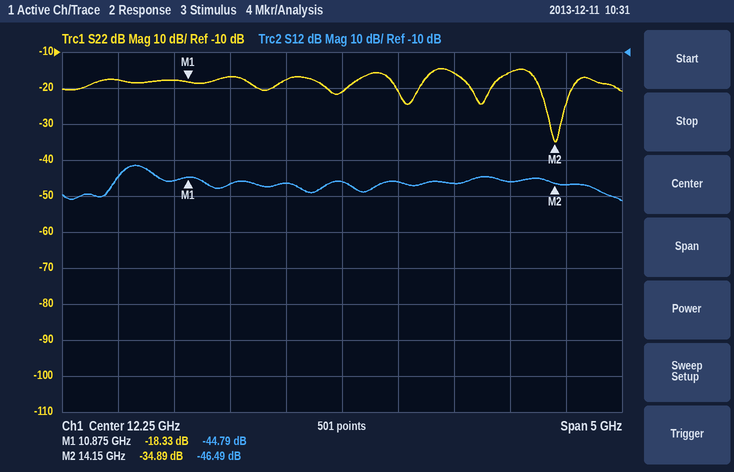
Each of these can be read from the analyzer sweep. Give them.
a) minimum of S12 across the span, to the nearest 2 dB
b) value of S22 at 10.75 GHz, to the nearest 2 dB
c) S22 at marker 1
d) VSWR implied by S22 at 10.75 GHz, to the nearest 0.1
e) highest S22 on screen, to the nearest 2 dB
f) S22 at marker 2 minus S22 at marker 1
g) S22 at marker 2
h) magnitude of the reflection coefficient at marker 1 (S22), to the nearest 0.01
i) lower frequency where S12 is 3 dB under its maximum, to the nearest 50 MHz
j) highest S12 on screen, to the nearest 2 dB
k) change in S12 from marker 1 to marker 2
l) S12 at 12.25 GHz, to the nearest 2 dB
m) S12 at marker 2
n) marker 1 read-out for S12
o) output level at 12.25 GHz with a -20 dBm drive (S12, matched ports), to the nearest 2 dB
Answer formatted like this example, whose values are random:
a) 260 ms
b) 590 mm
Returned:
a) -52 dB
b) -18 dB
c) -18.33 dB
d) 1.3
e) -14 dB
f) -16.56 dB
g) -34.89 dB
h) 0.12
i) 10.25 GHz
j) -42 dB
k) -1.70 dB
l) -46 dB
m) -46.49 dB
n) -44.79 dB
o) -66 dBm
